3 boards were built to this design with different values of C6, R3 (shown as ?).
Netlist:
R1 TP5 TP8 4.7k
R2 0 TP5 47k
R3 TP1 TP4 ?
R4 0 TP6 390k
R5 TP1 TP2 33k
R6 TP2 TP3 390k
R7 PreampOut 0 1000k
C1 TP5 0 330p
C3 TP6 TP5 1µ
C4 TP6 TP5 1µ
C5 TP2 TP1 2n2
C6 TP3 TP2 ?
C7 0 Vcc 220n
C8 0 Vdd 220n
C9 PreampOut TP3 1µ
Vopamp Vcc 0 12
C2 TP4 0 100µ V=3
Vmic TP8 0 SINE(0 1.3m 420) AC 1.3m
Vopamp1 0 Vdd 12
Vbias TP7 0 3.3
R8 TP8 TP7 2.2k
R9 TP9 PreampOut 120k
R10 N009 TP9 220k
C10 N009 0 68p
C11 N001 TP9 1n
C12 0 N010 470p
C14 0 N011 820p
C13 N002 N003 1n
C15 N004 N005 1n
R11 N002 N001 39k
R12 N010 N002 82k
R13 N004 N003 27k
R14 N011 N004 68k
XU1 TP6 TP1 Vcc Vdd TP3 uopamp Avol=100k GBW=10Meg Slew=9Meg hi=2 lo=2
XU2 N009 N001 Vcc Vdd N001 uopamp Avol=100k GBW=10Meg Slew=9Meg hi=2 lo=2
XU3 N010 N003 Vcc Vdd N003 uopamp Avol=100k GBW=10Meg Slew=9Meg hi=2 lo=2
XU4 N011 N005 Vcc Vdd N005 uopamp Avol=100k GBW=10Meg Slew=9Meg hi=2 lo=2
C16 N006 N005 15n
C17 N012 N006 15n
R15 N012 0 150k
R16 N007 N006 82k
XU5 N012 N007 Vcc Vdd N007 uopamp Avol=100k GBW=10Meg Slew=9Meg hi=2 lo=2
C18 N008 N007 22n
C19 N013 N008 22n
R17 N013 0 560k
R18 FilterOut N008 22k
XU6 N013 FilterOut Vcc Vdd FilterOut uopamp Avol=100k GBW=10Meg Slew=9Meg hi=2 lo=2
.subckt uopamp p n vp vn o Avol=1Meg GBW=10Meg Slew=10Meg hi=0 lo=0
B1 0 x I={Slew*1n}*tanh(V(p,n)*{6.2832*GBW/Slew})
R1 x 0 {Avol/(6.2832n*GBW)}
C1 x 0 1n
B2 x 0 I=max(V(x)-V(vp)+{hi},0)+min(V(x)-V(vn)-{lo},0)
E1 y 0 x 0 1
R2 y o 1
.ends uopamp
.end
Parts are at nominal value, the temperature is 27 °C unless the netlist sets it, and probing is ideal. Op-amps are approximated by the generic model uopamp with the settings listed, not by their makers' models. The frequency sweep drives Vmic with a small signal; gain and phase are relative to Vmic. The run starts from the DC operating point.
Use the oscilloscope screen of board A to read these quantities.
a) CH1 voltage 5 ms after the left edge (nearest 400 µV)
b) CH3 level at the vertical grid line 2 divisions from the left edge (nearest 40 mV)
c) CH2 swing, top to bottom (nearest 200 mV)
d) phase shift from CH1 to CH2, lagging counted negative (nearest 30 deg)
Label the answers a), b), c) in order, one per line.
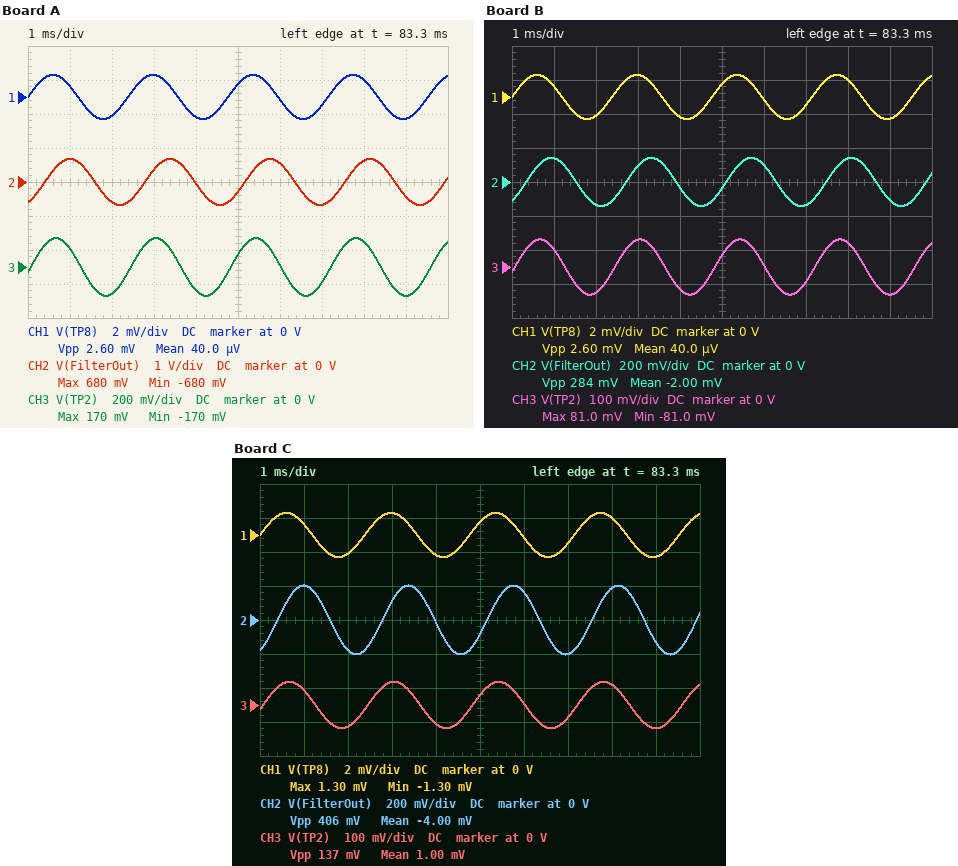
a) 800 µV
b) -160 mV
c) 1.4 V
d) -60 deg
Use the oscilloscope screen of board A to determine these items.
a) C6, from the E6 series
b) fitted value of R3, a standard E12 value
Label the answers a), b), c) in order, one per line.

a) 3.3 nF
b) 220 Ω
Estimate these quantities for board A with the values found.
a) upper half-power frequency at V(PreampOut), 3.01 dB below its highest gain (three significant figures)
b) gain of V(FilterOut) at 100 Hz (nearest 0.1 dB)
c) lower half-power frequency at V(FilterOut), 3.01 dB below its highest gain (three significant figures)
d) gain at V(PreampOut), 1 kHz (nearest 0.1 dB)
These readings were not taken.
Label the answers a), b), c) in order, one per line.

a) 139 Hz
b) 63.4 dB
c) 60.8 Hz
d) 48.7 dB
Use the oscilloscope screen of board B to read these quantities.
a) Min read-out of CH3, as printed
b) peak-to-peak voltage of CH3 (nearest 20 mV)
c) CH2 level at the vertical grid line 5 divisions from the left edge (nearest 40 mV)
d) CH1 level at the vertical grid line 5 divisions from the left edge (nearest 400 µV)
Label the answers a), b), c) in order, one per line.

a) -81.0 mV
b) 160 mV
c) -40 mV
d) 800 µV
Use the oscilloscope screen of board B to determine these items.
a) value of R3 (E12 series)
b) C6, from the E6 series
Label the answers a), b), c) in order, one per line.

a) 470 Ω
b) 10 nF
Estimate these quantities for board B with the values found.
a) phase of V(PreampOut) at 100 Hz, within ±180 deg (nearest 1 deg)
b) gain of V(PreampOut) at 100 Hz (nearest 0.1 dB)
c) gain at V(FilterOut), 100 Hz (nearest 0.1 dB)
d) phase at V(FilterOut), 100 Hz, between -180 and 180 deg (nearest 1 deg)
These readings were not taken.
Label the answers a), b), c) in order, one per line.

a) -55 deg
b) 49.9 dB
c) 50.9 dB
d) 50 deg
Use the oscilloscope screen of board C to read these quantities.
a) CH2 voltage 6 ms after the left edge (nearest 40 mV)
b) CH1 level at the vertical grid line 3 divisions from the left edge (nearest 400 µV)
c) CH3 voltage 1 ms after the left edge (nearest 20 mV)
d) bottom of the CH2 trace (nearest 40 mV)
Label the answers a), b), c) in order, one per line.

a) 160 mV
b) 1.2 mV
c) 40 mV
d) -200 mV
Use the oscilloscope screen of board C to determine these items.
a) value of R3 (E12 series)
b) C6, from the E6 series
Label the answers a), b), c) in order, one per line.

a) 560 Ω
b) 4.7 nF
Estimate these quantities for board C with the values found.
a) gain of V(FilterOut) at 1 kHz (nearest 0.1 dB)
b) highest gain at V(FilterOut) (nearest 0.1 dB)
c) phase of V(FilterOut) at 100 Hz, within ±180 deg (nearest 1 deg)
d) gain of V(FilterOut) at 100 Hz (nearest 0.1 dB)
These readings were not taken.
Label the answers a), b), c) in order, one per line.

a) 38.9 dB
b) 55.8 dB
c) 63 deg
d) 54.0 dB
